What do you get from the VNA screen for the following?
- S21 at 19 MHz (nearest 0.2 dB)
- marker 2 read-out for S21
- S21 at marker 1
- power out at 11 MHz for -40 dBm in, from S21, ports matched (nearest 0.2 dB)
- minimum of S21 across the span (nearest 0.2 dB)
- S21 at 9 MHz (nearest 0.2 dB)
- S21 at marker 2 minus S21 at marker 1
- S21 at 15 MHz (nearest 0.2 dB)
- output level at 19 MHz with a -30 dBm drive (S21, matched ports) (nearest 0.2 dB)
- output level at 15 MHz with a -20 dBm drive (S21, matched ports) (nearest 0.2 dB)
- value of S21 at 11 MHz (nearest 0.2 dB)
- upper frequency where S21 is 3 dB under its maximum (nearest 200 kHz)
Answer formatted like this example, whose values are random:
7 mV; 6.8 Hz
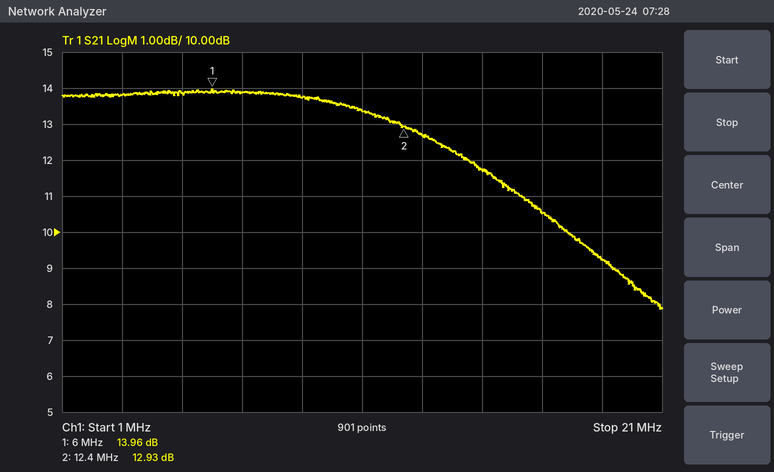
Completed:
9.2 dB; 12.93 dB; 13.96 dB; -26.6 dBm; 7.8 dB; 13.8 dB; -1.03 dB; 11.8 dB; -20.8 dBm; -8.2 dBm; 13.4 dB; 16.4 MHz
